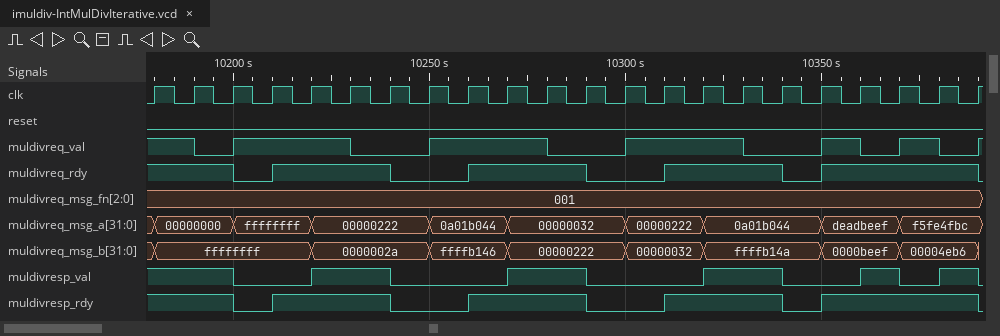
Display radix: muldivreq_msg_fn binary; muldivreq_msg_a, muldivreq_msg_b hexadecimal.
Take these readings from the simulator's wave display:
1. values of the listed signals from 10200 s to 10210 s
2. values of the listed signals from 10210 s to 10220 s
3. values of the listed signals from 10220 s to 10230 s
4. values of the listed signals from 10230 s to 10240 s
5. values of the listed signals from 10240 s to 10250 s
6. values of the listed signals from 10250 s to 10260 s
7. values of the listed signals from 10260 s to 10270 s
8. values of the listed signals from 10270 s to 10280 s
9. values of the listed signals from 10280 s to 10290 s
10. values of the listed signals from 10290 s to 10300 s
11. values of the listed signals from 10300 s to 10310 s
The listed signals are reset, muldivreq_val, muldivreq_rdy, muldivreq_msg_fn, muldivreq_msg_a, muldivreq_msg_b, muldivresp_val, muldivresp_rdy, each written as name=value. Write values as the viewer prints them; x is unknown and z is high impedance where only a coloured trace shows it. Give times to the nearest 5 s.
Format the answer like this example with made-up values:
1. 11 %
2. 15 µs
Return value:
1. reset=0, muldivreq_val=1, muldivreq_rdy=0, muldivreq_msg_fn=001, muldivreq_msg_a=ffffffff, muldivreq_msg_b=ffffffff, muldivresp_val=0, muldivresp_rdy=0
2. reset=0, muldivreq_val=1, muldivreq_rdy=1, muldivreq_msg_fn=001, muldivreq_msg_a=ffffffff, muldivreq_msg_b=ffffffff, muldivresp_val=0, muldivresp_rdy=1
3. reset=0, muldivreq_val=1, muldivreq_rdy=1, muldivreq_msg_fn=001, muldivreq_msg_a=00000222, muldivreq_msg_b=0000002a, muldivresp_val=1, muldivresp_rdy=1
4. reset=0, muldivreq_val=0, muldivreq_rdy=1, muldivreq_msg_fn=001, muldivreq_msg_a=00000222, muldivreq_msg_b=0000002a, muldivresp_val=1, muldivresp_rdy=1
5. reset=0, muldivreq_val=0, muldivreq_rdy=0, muldivreq_msg_fn=001, muldivreq_msg_a=00000222, muldivreq_msg_b=0000002a, muldivresp_val=0, muldivresp_rdy=0
6. reset=0, muldivreq_val=1, muldivreq_rdy=0, muldivreq_msg_fn=001, muldivreq_msg_a=0a01b044, muldivreq_msg_b=ffffb146, muldivresp_val=0, muldivresp_rdy=0
7. reset=0, muldivreq_val=1, muldivreq_rdy=1, muldivreq_msg_fn=001, muldivreq_msg_a=0a01b044, muldivreq_msg_b=ffffb146, muldivresp_val=0, muldivresp_rdy=1
8. reset=0, muldivreq_val=1, muldivreq_rdy=1, muldivreq_msg_fn=001, muldivreq_msg_a=00000032, muldivreq_msg_b=00000222, muldivresp_val=1, muldivresp_rdy=1
9. reset=0, muldivreq_val=0, muldivreq_rdy=1, muldivreq_msg_fn=001, muldivreq_msg_a=00000032, muldivreq_msg_b=00000222, muldivresp_val=1, muldivresp_rdy=1
10. reset=0, muldivreq_val=0, muldivreq_rdy=0, muldivreq_msg_fn=001, muldivreq_msg_a=00000032, muldivreq_msg_b=00000222, muldivresp_val=0, muldivresp_rdy=0
11. reset=0, muldivreq_val=1, muldivreq_rdy=0, muldivreq_msg_fn=001, muldivreq_msg_a=00000222, muldivreq_msg_b=00000032, muldivresp_val=0, muldivresp_rdy=0
